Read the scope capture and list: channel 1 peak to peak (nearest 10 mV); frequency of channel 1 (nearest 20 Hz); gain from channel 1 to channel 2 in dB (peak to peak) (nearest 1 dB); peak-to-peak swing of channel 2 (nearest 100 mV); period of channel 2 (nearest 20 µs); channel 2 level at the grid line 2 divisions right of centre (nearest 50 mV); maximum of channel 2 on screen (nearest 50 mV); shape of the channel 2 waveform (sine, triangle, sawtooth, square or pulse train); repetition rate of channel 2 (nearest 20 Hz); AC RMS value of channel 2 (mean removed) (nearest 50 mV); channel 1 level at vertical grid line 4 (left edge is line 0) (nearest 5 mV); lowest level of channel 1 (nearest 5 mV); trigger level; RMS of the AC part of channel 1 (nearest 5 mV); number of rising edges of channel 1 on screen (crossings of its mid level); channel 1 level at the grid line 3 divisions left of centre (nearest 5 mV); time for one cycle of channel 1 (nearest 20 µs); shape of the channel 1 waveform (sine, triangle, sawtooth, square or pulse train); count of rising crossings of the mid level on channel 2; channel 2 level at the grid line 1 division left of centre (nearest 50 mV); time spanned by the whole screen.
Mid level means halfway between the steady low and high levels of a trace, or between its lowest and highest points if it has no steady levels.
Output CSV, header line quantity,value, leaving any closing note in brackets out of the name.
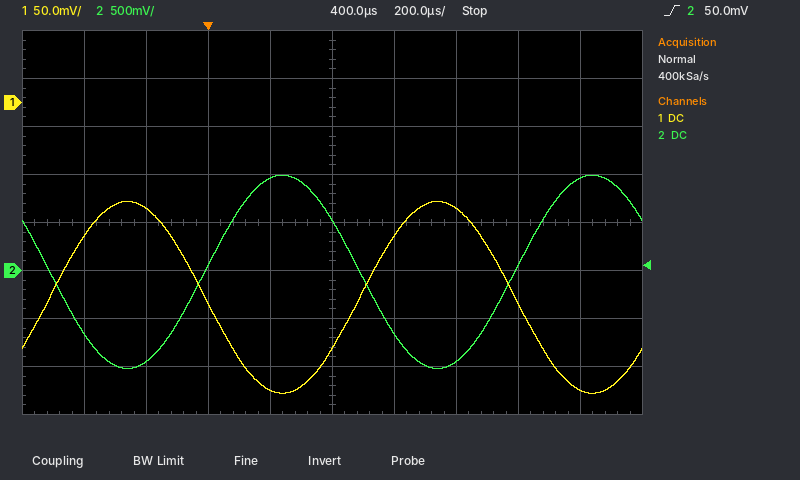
quantity,value
channel 1 peak to peak,200 mV
frequency of channel 1,1.00 kHz
gain from channel 1 to channel 2 in dB (peak to peak),20 dB
peak-to-peak swing of channel 2,2.00 V
period of channel 2,1.00 ms
channel 2 level at the grid line 2 divisions right of centre,-950 mV
maximum of channel 2 on screen,1.00 V
shape of the channel 2 waveform,sine
repetition rate of channel 2,1.00 kHz
AC RMS value of channel 2 (mean removed),700 mV
channel 1 level at vertical grid line 4 (left edge is line 0),-300 mV
lowest level of channel 1,-305 mV
trigger level,50.0 mV
RMS of the AC part of channel 1,70 mV
number of rising edges of channel 1 on screen,2
channel 1 level at the grid line 3 divisions left of centre,-110 mV
time for one cycle of channel 1,1.00 ms
shape of the channel 1 waveform,sine
count of rising crossings of the mid level on channel 2,2
channel 2 level at the grid line 1 division left of centre,950 mV
time spanned by the whole screen,2 ms
